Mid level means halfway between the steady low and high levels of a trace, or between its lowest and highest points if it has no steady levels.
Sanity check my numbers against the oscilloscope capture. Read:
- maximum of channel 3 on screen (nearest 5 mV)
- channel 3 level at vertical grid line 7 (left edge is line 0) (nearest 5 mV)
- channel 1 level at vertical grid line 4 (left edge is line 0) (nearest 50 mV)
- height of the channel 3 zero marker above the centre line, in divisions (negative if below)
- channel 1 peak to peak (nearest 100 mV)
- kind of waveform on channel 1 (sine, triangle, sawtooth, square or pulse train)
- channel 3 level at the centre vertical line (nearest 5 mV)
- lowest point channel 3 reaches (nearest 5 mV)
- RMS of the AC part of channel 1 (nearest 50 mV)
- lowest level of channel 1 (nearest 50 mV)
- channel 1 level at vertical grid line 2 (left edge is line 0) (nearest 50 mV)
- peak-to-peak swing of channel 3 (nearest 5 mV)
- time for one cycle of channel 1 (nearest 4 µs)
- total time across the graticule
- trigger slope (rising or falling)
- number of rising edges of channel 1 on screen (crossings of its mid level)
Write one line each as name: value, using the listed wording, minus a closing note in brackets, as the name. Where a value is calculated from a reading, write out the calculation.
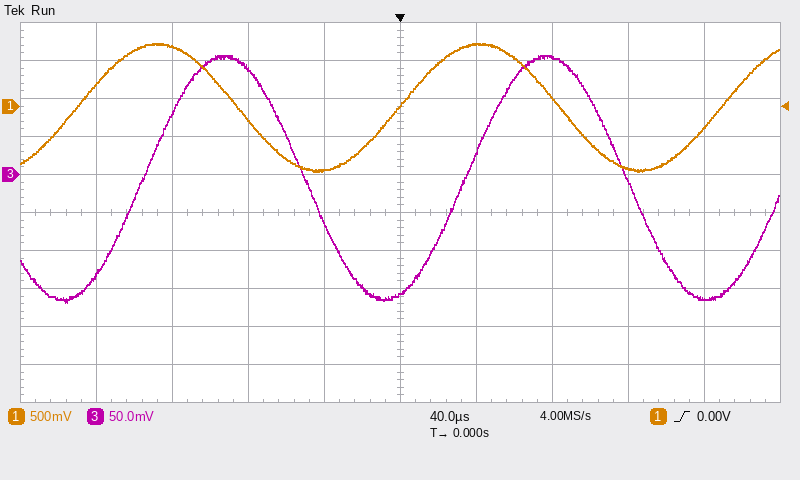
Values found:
maximum of channel 3 on screen: 155 mV
channel 3 level at vertical grid line 7 (left edge is line 0): 155 mV
channel 1 level at vertical grid line 4 (left edge is line 0): -850 mV
height of the channel 3 zero marker above the centre line, in divisions: +1.0 div
channel 1 peak to peak: 1.70 V
kind of waveform on channel 1: sine
channel 3 level at the centre vertical line: -155 mV
lowest point channel 3 reaches: -170 mV
RMS of the AC part of channel 1: 1.70 V / (2√2) ≈ 601 mV, so 600 mV to the nearest 50 mV
lowest level of channel 1: -850 mV
channel 1 level at vertical grid line 2 (left edge is line 0): 800 mV
peak-to-peak swing of channel 3: 155 mV − (-170 mV) = 325 mV
time for one cycle of channel 1: 168 µs
total time across the graticule: 400 µs
trigger slope: rising
number of rising edges of channel 1 on screen: 3
